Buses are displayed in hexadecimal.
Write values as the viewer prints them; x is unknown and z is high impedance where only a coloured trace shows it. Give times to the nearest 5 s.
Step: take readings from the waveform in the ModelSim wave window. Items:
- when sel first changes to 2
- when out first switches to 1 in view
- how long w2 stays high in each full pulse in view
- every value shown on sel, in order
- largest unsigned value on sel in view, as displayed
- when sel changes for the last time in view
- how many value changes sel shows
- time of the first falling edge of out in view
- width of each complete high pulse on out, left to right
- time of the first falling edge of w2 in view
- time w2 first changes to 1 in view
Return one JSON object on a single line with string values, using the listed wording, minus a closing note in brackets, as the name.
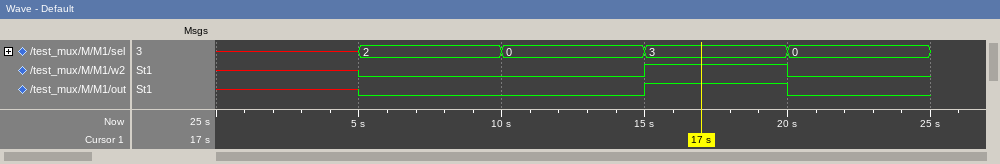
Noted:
{"when sel first changes to 2": "5 s", "when out first switches to 1 in view": "15 s", "how long w2 stays high in each full pulse in view": "5 s", "every value shown on sel, in order": "x, 2, 0, 3, 0", "largest unsigned value on sel in view, as displayed": "3", "when sel changes for the last time in view": "20 s", "how many value changes sel shows": "4", "time of the first falling edge of out in view": "20 s", "width of each complete high pulse on out, left to right": "5 s", "time of the first falling edge of w2 in view": "20 s", "time w2 first changes to 1 in view": "15 s"}
